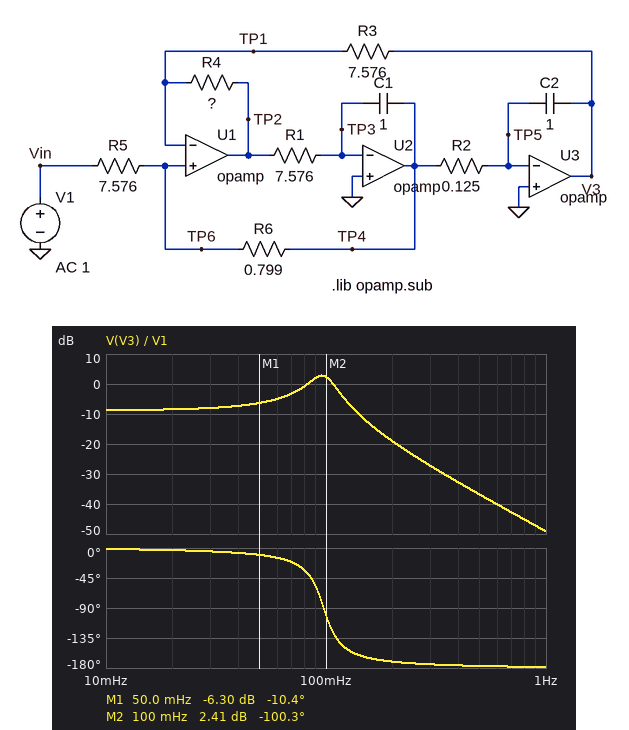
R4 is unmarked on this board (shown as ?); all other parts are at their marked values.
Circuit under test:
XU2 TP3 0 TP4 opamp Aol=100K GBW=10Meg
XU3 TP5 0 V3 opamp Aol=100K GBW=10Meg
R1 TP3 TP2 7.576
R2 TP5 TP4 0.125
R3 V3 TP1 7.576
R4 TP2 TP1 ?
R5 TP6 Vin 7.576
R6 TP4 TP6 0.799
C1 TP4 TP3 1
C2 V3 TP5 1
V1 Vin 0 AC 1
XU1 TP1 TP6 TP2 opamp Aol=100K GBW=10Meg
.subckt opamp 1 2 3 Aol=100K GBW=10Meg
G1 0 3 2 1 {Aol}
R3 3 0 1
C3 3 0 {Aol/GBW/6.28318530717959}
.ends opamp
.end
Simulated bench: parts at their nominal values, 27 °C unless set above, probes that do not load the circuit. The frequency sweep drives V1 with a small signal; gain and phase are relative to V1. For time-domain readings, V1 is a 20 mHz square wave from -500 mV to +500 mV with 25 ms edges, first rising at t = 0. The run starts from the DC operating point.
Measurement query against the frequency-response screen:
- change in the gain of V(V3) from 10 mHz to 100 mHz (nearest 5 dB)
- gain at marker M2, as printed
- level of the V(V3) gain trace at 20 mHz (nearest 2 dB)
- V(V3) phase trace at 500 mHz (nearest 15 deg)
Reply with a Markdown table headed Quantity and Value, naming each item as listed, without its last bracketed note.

| Quantity | Value |
|---|---|
| change in the gain of V(V3) from 10 mHz to 100 mHz | 10 dB |
| gain at marker M2, as printed | 2.41 dB |
| level of the V(V3) gain trace at 20 mHz | -8 dB |
| V(V3) phase trace at 500 mHz | -180 deg |
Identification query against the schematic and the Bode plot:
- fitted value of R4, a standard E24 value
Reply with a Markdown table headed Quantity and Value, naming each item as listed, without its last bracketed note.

| Quantity | Value |
|---|---|
| fitted value of R4, a standard E24 value | 2.7 Ω |
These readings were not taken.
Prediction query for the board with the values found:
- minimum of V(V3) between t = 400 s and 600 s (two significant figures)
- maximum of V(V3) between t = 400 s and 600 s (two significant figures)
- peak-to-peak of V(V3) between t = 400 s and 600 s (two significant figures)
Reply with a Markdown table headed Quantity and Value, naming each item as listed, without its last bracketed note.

| Quantity | Value |
|---|---|
| minimum of V(V3) between t = 400 s and 600 s | -450 mV |
| maximum of V(V3) between t = 400 s and 600 s | 450 mV |
| peak-to-peak of V(V3) between t = 400 s and 600 s | 900 mV |
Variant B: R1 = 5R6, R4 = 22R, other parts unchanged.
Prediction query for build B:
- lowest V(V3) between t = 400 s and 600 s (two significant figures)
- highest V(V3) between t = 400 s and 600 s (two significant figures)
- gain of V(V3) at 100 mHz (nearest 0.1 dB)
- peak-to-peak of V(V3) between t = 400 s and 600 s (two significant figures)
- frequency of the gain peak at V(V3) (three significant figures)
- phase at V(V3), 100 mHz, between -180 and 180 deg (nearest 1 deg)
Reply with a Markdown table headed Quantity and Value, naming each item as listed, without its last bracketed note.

| Quantity | Value |
|---|---|
| lowest V(V3) between t = 400 s and 600 s | -140 mV |
| highest V(V3) between t = 400 s and 600 s | 140 mV |
| gain of V(V3) at 100 mHz | -17.0 dB |
| peak-to-peak of V(V3) between t = 400 s and 600 s | 290 mV |
| frequency of the gain peak at V(V3) | 316 mHz |
| phase at V(V3), 100 mHz, between -180 and 180 deg | -6 deg |
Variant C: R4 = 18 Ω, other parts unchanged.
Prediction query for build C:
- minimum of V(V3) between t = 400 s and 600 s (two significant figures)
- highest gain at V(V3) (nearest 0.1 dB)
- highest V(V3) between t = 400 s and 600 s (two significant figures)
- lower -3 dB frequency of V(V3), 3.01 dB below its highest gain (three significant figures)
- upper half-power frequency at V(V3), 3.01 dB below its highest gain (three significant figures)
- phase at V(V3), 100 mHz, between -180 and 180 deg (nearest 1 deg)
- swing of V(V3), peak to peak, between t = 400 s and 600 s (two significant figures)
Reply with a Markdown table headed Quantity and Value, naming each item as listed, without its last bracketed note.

| Quantity | Value |
|---|---|
| minimum of V(V3) between t = 400 s and 600 s | -160 mV |
| highest gain at V(V3) | -5.4 dB |
| highest V(V3) between t = 400 s and 600 s | 160 mV |
| lower -3 dB frequency of V(V3), 3.01 dB below its highest gain | 213 mHz |
| upper half-power frequency at V(V3), 3.01 dB below its highest gain | 278 mHz |
| phase at V(V3), 100 mHz, between -180 and 180 deg | -7 deg |
| swing of V(V3), peak to peak, between t = 400 s and 600 s | 320 mV |
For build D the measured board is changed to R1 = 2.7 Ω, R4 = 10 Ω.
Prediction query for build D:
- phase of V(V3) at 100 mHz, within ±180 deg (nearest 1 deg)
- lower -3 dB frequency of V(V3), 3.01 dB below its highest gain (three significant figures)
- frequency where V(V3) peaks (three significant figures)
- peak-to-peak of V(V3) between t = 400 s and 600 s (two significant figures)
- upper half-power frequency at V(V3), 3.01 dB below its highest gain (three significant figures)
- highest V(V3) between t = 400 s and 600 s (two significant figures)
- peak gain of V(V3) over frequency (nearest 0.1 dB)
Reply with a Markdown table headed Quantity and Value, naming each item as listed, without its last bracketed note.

| Quantity | Value |
|---|---|
| phase of V(V3) at 100 mHz, within ±180 deg | -8 deg |
| lower -3 dB frequency of V(V3), 3.01 dB below its highest gain | 231 mHz |
| frequency where V(V3) peaks | 302 mHz |
| peak-to-peak of V(V3) between t = 400 s and 600 s | 350 mV |
| upper half-power frequency at V(V3), 3.01 dB below its highest gain | 360 mHz |
| highest V(V3) between t = 400 s and 600 s | 170 mV |
| peak gain of V(V3) over frequency | -7.2 dB |
